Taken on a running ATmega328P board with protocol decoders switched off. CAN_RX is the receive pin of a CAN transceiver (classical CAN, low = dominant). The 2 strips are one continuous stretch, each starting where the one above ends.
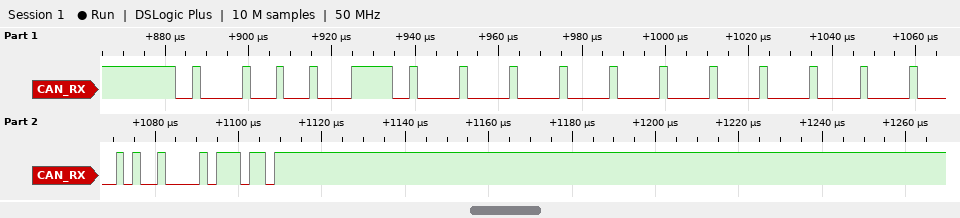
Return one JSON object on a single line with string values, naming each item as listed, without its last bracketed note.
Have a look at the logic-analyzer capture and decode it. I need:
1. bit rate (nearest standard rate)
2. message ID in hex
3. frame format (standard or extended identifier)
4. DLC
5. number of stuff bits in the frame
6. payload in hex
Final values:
{"bit rate": "500 kbit/s", "message ID in hex": "0x201", "frame format": "standard", "DLC": "8", "number of stuff bits in the frame": "13", "payload in hex": "7D 00 00 00 00 00 00 00"}
